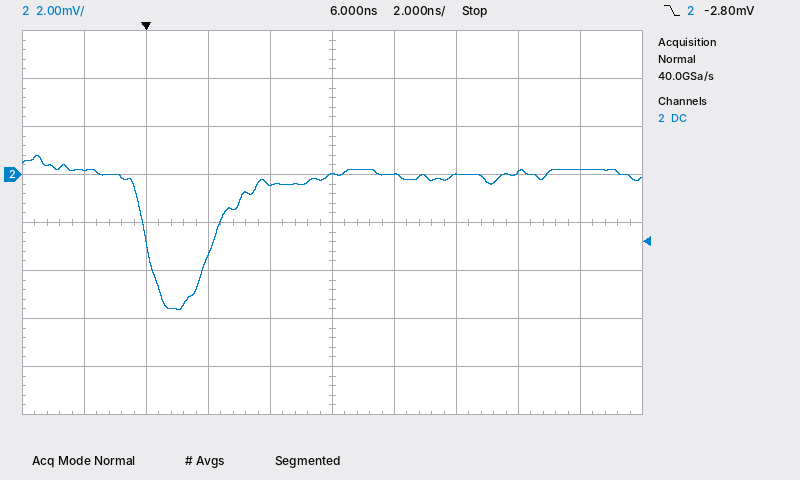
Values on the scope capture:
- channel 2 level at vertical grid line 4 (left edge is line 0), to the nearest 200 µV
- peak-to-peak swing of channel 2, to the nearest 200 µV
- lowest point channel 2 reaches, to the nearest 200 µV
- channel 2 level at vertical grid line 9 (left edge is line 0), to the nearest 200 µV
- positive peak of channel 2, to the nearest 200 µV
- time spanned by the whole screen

-400 µV
6.4 mV
-5.6 mV
200 µV
800 µV
20 ns
